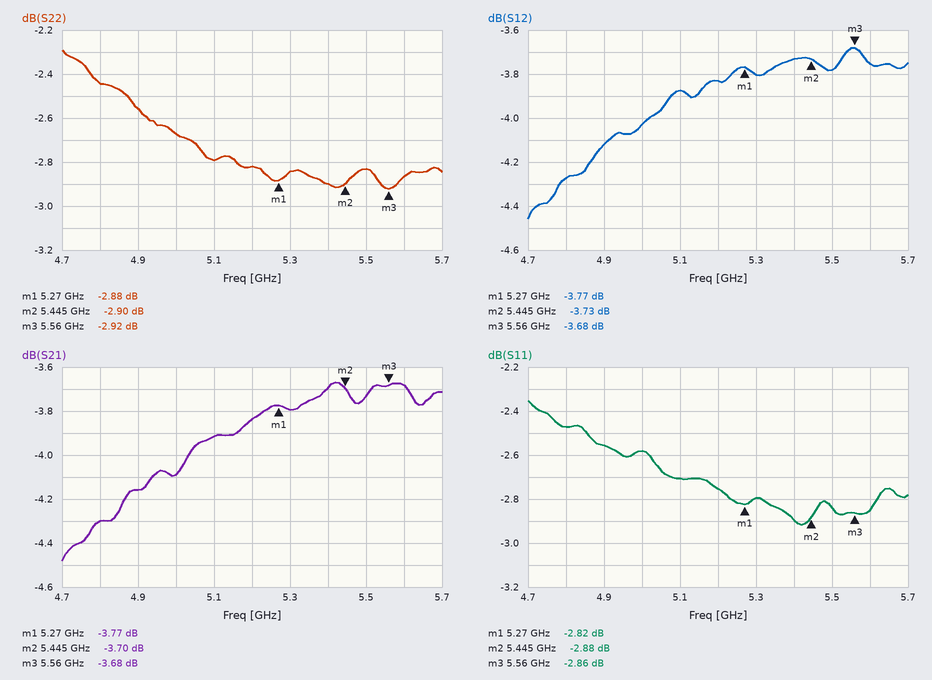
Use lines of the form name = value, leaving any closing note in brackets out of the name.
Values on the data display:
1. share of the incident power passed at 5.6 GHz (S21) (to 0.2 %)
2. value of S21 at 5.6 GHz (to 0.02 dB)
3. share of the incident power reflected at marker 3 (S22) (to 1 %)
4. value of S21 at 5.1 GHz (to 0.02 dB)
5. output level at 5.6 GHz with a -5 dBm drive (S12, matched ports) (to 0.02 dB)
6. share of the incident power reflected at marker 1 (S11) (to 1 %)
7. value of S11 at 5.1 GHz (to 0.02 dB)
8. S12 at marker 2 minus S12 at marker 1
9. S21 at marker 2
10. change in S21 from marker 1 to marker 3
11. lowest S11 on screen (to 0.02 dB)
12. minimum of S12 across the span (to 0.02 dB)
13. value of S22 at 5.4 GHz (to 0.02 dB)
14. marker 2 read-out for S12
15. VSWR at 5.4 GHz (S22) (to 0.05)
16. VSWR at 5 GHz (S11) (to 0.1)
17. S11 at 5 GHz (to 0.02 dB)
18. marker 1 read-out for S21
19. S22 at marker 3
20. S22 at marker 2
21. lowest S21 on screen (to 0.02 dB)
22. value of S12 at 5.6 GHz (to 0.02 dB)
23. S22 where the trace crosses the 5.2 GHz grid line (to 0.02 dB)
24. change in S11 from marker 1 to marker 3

share of the incident power passed at 5.6 GHz (S21) = 42.8 %
value of S21 at 5.6 GHz = -3.68 dB
share of the incident power reflected at marker 3 (S22) = 51 %
value of S21 at 5.1 GHz = -3.92 dB
output level at 5.6 GHz with a -5 dBm drive (S12, matched ports) = -8.76 dBm
share of the incident power reflected at marker 1 (S11) = 52 %
value of S11 at 5.1 GHz = -2.70 dB
S12 at marker 2 minus S12 at marker 1 = 0.04 dB
S21 at marker 2 = -3.70 dB
change in S21 from marker 1 to marker 3 = 0.09 dB
lowest S11 on screen = -2.92 dB
minimum of S12 across the span = -4.46 dB
value of S22 at 5.4 GHz = -2.90 dB
marker 2 read-out for S12 = -3.73 dB
VSWR at 5.4 GHz (S22) = 6.05
VSWR at 5 GHz (S11) = 6.8
S11 at 5 GHz = -2.58 dB
marker 1 read-out for S21 = -3.77 dB
S22 at marker 3 = -2.92 dB
S22 at marker 2 = -2.90 dB
lowest S21 on screen = -4.48 dB
value of S12 at 5.6 GHz = -3.76 dB
S22 where the trace crosses the 5.2 GHz grid line = -2.82 dB
change in S11 from marker 1 to marker 3 = -0.04 dB
